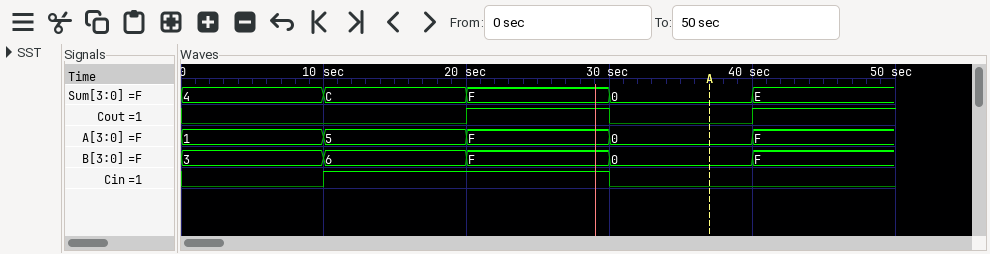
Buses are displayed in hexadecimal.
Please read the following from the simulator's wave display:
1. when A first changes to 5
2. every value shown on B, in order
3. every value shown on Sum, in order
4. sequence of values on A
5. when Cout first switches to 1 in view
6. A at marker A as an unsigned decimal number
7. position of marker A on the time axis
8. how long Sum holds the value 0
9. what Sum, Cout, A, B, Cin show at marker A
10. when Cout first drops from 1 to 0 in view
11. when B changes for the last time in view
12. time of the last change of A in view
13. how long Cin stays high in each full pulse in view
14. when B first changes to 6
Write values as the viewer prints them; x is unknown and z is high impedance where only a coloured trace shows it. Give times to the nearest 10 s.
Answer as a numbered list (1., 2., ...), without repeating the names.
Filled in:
1. 10 s
2. 3, 6, F, 0, F
3. 4, C, F, 0, E
4. 1, 5, F, 0, F
5. 20 s
6. 0
7. 40 s
8. 10 s
9. Sum=0, Cout=0, A=0, B=0, Cin=0
10. 30 s
11. 40 s
12. 40 s
13. 20 s
14. 10 s
